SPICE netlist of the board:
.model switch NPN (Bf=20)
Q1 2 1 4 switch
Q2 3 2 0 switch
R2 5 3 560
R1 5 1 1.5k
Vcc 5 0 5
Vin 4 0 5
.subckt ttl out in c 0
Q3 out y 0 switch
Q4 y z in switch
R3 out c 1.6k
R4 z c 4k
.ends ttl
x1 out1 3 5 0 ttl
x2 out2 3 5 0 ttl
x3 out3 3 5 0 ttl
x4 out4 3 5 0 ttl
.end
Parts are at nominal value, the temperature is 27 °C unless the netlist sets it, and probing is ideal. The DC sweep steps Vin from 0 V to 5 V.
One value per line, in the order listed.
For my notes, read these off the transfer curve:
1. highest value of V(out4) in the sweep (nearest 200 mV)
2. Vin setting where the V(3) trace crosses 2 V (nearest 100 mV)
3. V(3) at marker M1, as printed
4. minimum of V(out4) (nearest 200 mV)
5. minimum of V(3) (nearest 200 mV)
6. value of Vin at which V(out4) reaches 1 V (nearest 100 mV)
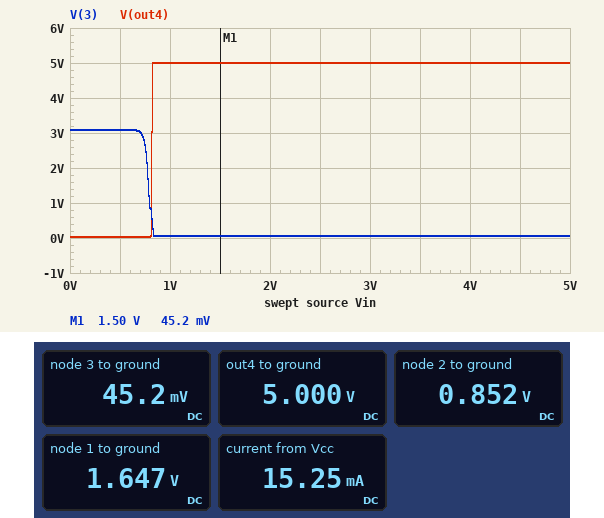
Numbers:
5.0 V
800 mV
45.2 mV
0 V
0 V
800 mV
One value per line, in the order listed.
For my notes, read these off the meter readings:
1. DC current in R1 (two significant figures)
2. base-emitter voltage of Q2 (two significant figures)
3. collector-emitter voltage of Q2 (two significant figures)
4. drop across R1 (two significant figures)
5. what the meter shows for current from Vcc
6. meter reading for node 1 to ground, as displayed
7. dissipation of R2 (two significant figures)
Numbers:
2.2 mA
850 mV
45 mV
3.4 V
15.25 mA
1.647 V
44 mW
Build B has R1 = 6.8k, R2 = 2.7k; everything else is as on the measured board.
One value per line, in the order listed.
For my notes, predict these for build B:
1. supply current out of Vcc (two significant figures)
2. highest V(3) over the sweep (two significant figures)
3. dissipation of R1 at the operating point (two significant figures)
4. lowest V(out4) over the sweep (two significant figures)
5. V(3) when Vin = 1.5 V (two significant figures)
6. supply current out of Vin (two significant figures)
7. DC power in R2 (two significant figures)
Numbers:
6.5 mA
830 mV
1.7 mW
42 mV
63 mV
500 µA
9.0 mW
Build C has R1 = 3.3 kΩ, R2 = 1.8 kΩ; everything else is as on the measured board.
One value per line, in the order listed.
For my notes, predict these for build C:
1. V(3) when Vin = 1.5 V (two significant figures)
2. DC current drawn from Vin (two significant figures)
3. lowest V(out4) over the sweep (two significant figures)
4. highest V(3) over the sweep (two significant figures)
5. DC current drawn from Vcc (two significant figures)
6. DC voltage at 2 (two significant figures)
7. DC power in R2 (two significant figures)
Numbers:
48 mV
1.0 mA
40 mV
850 mV
7.9 mA
830 mV
14 mW
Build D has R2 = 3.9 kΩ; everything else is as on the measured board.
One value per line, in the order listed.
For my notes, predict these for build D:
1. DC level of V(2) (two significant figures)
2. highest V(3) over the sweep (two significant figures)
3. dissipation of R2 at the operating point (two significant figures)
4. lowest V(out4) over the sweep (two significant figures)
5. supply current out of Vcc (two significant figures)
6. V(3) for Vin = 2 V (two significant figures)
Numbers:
840 mV
830 mV
6.3 mW
44 mV
7.7 mA
32 mV
